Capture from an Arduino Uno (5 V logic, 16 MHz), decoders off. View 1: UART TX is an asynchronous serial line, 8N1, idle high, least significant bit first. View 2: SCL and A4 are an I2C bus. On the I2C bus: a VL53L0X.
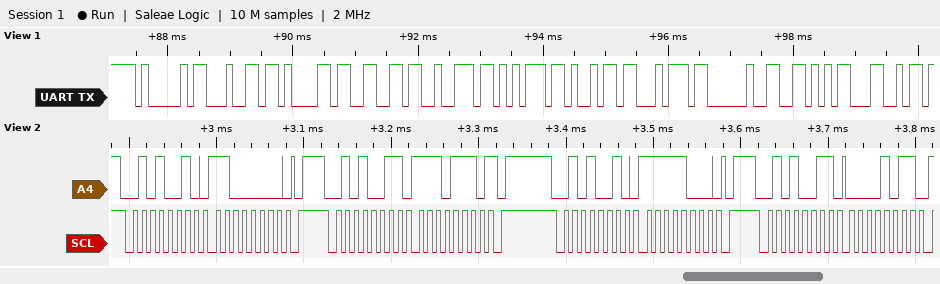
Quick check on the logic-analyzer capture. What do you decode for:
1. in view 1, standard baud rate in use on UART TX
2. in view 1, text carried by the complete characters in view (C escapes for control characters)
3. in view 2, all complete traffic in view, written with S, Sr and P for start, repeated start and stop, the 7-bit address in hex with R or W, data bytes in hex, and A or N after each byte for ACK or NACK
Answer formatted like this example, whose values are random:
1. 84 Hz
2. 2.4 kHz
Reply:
1. 9600 baud
2. "Adafruit VL"
3. S 29W A C0 A P S 29R A EE N P S 29W A F8 A P S 29R A 0B A
